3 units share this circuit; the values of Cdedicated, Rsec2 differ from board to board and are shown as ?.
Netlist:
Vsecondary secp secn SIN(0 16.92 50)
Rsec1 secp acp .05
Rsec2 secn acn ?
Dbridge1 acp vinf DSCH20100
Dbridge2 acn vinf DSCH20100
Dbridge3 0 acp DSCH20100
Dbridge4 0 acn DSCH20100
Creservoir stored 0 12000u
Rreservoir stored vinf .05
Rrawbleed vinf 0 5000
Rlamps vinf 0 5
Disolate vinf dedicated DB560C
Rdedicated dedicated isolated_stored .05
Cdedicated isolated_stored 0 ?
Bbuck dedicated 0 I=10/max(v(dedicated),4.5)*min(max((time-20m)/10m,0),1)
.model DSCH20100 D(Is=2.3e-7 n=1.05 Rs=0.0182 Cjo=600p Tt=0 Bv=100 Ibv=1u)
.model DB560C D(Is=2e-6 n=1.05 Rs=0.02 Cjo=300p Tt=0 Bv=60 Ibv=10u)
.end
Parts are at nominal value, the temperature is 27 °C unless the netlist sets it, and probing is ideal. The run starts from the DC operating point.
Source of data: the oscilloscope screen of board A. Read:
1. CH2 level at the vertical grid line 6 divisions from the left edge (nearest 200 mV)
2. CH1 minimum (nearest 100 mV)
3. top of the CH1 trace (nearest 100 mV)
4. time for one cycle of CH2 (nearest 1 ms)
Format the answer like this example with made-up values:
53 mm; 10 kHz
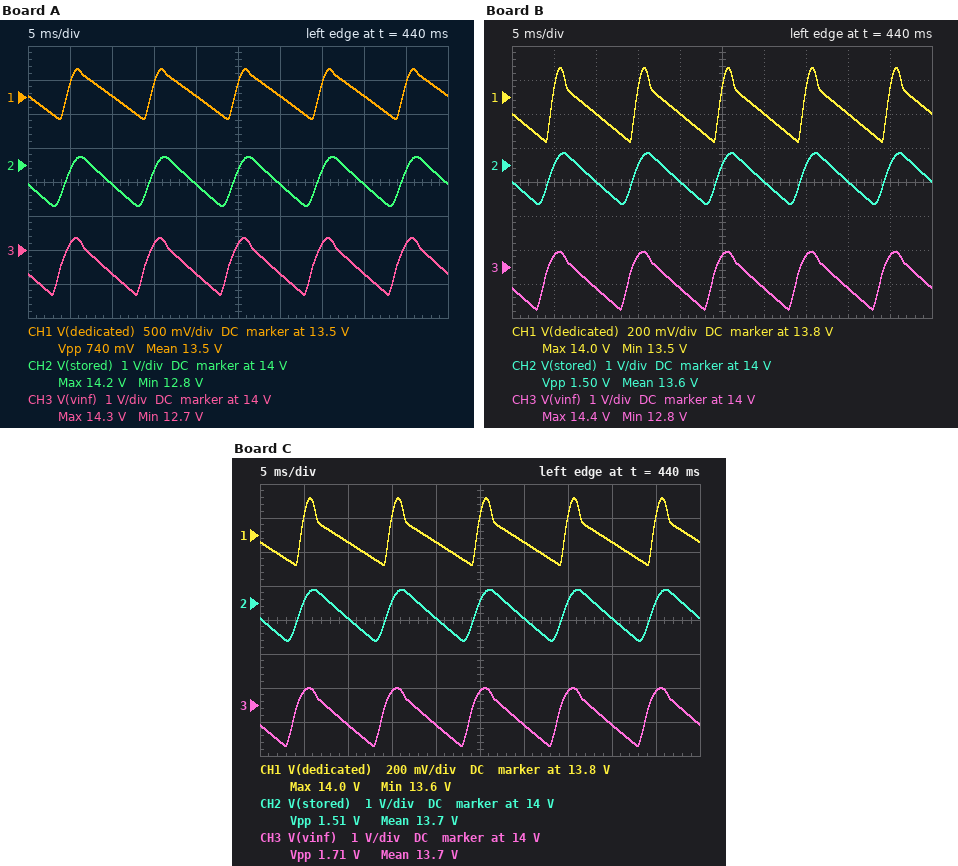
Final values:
13.4 V; 13.2 V; 13.9 V; 10 ms
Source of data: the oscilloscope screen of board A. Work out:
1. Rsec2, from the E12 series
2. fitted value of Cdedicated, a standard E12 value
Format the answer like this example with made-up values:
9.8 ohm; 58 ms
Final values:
0.039 Ω; 8.2 mF
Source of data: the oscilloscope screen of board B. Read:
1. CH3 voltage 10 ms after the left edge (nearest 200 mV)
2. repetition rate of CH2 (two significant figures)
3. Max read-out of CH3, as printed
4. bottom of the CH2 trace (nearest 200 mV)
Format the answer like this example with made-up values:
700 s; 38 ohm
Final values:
13.4 V; 100 Hz; 14.4 V; 12.8 V
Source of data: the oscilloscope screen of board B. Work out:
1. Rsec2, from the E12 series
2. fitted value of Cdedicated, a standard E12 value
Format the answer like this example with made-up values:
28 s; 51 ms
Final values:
0.027 Ω; 18 mF
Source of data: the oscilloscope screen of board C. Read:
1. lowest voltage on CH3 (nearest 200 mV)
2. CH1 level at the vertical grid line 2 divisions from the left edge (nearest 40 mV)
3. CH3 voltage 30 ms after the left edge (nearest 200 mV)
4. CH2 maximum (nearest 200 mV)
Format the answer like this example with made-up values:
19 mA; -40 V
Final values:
12.8 V; 13.76 V; 13.4 V; 14.4 V
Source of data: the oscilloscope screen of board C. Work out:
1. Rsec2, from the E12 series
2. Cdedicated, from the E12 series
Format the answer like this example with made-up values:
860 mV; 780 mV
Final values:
0.022 Ω; 22 mF
